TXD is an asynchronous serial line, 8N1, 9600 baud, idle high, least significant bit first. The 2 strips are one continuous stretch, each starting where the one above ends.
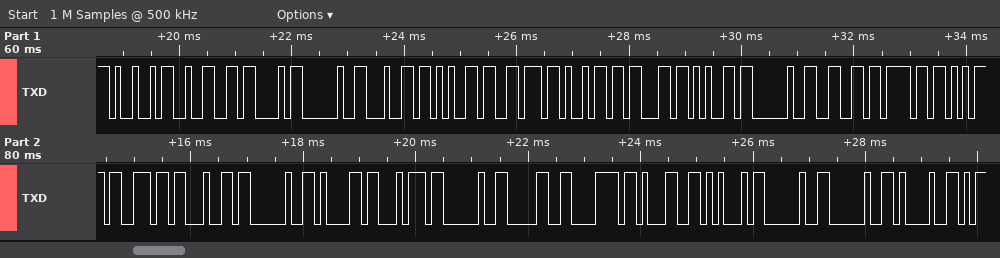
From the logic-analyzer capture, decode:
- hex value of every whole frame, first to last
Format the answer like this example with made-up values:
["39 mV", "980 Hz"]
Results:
["49 32 43 20 64 65 76 69 63 65 20 66 6F 75 6E 64 20 61 74 20 30 78 31 45 20 20 21"]
